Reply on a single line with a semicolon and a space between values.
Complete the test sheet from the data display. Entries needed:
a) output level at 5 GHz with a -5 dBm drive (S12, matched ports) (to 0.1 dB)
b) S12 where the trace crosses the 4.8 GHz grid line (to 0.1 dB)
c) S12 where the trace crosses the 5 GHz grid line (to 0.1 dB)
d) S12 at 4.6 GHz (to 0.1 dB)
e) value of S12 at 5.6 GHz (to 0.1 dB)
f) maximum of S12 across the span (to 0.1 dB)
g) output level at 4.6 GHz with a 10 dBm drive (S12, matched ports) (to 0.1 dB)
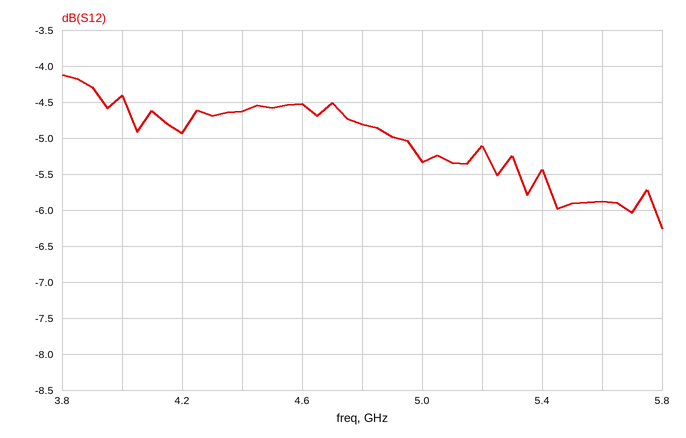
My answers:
-10.3 dBm; -4.8 dB; -5.3 dB; -4.5 dB; -5.9 dB; -4.1 dB; 5.5 dBm
